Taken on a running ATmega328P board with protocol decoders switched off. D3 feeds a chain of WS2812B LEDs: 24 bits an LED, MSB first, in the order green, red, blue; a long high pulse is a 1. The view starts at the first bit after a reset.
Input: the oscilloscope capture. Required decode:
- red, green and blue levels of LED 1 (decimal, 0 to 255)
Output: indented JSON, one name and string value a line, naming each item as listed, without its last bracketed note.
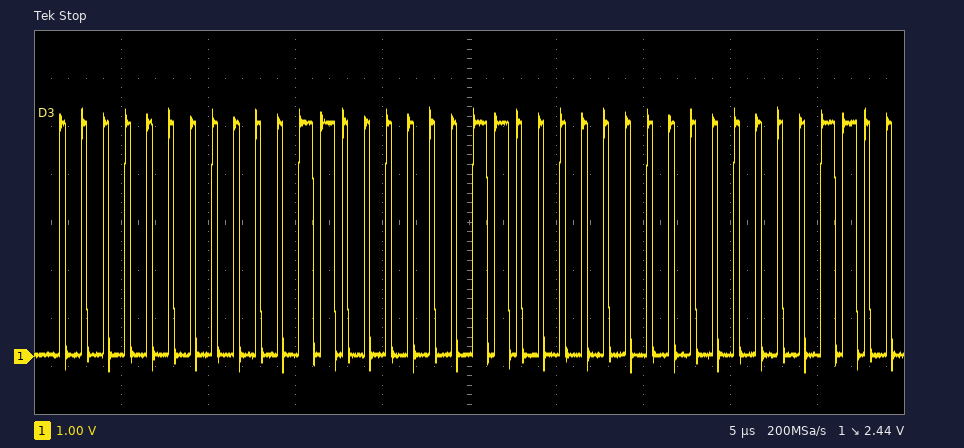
{
  "red, green and blue levels of LED 1": "24, 0, 24"
}
